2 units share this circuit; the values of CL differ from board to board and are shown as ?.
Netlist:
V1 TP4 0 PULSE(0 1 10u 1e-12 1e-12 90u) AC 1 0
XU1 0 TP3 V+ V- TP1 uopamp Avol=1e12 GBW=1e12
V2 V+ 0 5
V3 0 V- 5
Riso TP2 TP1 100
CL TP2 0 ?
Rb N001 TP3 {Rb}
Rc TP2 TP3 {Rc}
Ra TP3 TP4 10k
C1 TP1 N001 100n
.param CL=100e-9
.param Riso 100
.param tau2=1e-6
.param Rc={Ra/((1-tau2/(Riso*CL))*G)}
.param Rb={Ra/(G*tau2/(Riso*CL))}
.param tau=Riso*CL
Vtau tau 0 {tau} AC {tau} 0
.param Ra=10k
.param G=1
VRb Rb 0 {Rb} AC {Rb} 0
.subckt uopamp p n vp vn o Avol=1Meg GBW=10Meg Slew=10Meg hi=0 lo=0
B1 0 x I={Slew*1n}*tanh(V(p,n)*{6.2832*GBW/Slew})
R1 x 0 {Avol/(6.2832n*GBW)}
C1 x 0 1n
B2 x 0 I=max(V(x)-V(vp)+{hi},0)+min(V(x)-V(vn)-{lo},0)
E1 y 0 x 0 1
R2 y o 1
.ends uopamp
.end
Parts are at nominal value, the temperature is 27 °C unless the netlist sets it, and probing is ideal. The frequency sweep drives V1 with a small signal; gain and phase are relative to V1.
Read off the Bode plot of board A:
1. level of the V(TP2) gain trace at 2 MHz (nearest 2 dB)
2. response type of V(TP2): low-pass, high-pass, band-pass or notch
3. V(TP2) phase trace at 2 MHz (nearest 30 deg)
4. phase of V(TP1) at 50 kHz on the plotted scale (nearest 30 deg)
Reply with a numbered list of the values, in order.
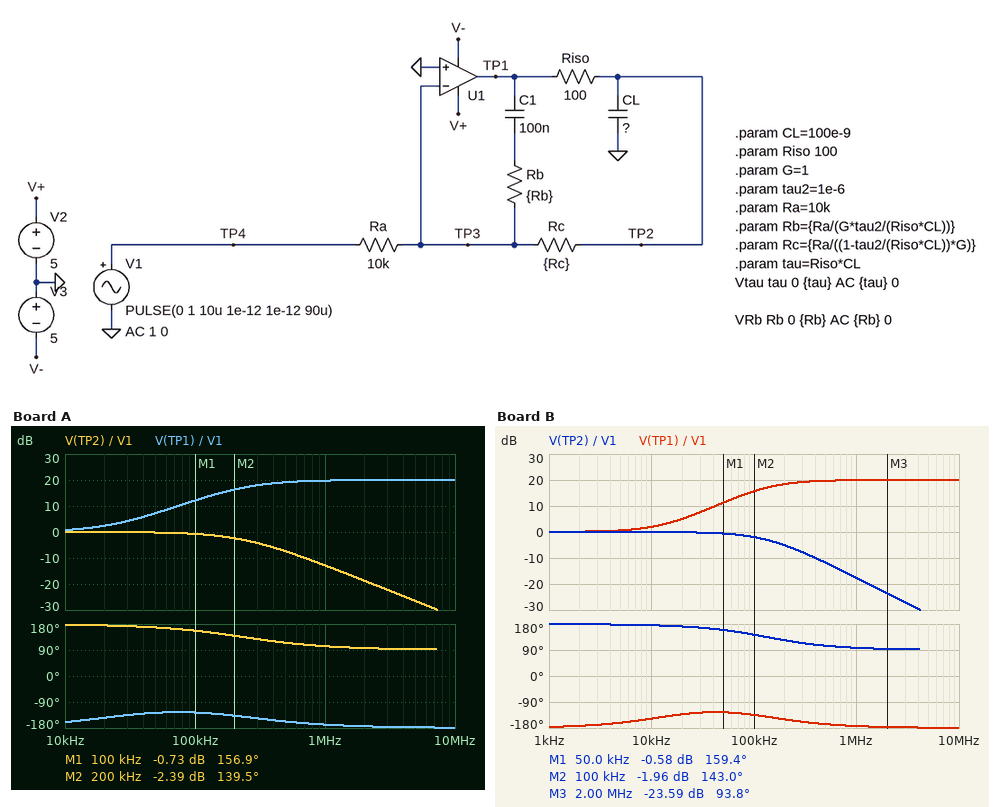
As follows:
1. -18 dB
2. low-pass
3. 90 deg
4. -120 deg
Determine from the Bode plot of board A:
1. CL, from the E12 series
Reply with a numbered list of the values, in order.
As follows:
1. 68 nF
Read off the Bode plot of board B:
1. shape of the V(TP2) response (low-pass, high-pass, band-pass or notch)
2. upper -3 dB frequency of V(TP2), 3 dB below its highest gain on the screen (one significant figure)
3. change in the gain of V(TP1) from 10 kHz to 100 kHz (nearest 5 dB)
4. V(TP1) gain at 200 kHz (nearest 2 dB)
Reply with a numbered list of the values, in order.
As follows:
1. low-pass
2. 100 kHz
3. 15 dB
4. 18 dB
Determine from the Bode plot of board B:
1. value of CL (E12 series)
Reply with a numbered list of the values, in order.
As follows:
1. 120 nF
